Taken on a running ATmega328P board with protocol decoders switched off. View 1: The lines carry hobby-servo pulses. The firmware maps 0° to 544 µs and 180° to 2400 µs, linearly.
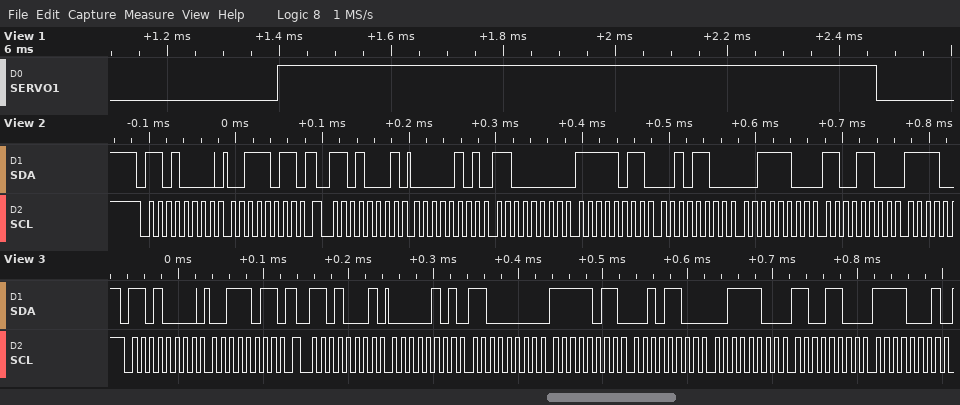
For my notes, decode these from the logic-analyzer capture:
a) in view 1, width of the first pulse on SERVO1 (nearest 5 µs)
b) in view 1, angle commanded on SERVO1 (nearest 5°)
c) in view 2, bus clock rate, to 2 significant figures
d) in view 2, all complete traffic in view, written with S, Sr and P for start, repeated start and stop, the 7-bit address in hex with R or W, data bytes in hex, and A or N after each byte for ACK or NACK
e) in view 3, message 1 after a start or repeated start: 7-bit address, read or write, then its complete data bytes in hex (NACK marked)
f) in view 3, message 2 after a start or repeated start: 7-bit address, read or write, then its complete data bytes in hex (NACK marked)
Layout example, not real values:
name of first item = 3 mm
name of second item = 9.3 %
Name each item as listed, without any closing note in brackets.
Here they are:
in view 1, width of the first pulse on SERVO1 = 1070 µs
in view 1, angle commanded on SERVO1 = 50°
in view 2, bus clock rate, to 2 significant figures = 100 kHz
in view 2, all complete traffic in view, written with S, Sr and P for start, repeated start and stop, the 7-bit address in hex with R or W, data bytes in hex, and A or N after each byte for ACK or NACK = S 68W A 3B A Sr 68R A 05 A C0 A FB A 2C A 3C A CC A
in view 3, message 1 after a start or repeated start: 7-bit address, read or write, then its complete data bytes in hex = 0x68 write: 3B
in view 3, message 2 after a start or repeated start: 7-bit address, read or write, then its complete data bytes in hex = 0x68 read: 05 C0 FB 2C 3C CC F1
